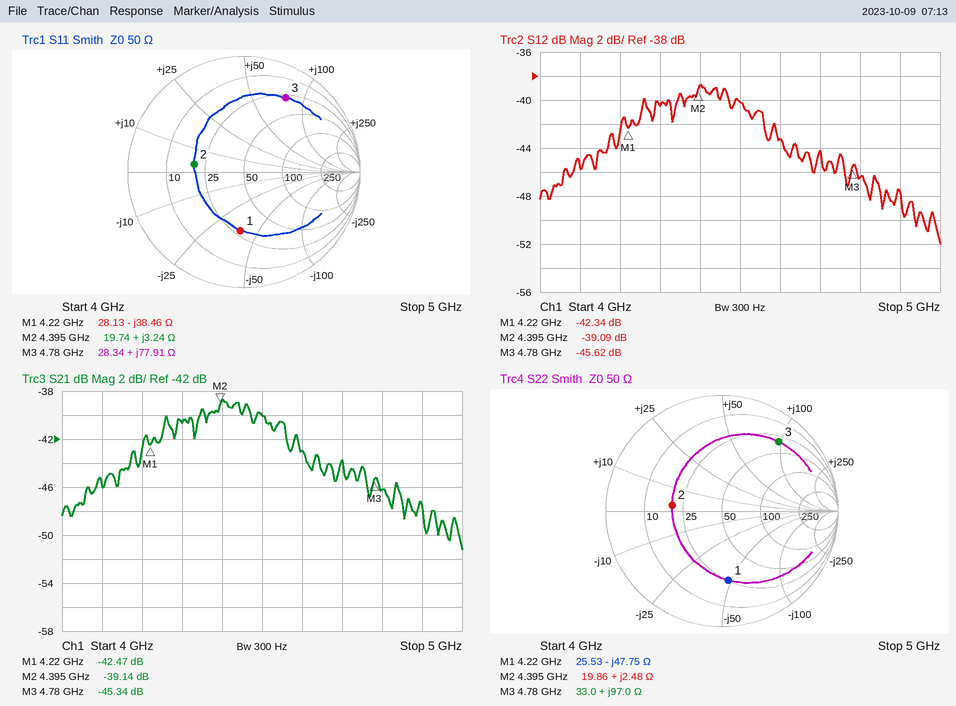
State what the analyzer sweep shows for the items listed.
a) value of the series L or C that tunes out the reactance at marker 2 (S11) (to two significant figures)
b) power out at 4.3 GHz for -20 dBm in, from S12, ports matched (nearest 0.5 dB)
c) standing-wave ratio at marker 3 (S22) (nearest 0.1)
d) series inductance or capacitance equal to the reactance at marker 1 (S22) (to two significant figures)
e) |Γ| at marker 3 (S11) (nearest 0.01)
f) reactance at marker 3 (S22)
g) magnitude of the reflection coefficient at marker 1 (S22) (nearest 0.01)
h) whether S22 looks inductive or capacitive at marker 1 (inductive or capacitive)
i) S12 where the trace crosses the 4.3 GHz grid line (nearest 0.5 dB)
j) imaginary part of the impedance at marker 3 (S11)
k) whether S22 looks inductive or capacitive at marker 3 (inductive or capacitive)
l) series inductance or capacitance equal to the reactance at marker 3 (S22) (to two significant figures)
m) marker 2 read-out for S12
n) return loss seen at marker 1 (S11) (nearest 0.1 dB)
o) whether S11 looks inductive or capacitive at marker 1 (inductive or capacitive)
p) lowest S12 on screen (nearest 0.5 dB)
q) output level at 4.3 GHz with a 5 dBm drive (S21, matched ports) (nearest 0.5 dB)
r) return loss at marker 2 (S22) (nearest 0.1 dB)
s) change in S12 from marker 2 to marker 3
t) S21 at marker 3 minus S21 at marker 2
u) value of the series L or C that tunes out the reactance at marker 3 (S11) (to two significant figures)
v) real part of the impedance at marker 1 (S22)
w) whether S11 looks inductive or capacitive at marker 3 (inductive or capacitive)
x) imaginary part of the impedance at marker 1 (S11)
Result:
11 pF
-60.5 dBm
7.7
790 fF
0.73
+97.0 Ω
0.60
capacitive
-40.5 dB
+77.91 Ω
inductive
3.2 nH
-39.09 dB
5.9 dB
capacitive
-52.0 dB
-35.5 dBm
7.3 dB
-6.53 dB
-6.20 dB
430 fF
25.53 Ω
inductive
-38.46 Ω
